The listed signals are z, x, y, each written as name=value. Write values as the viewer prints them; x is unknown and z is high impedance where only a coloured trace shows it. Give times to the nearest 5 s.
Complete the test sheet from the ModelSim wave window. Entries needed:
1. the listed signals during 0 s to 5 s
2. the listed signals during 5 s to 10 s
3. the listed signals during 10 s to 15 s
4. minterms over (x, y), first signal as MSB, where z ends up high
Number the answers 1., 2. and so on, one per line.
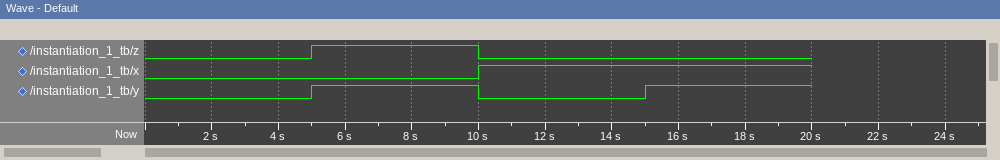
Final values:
1. z=0, x=0, y=0
2. z=1, x=0, y=1
3. z=0, x=1, y=0
4. 1
